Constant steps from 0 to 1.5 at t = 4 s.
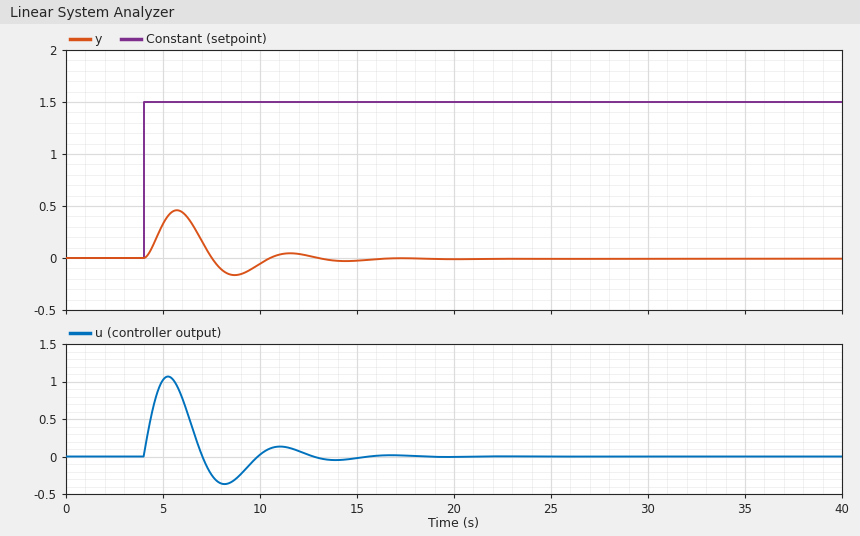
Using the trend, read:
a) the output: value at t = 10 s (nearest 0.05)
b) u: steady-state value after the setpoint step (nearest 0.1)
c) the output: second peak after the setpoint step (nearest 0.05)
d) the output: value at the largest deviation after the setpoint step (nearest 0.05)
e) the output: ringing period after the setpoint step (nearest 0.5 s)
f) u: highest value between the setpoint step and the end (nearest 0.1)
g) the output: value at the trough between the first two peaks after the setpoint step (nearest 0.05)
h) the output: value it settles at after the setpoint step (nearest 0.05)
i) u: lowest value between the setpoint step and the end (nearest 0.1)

-0.05
0.0
0.05
0.45
6.0 s
1.1
-0.15
0.00
-0.4
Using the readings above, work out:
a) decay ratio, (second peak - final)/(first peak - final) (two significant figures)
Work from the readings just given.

0.11
